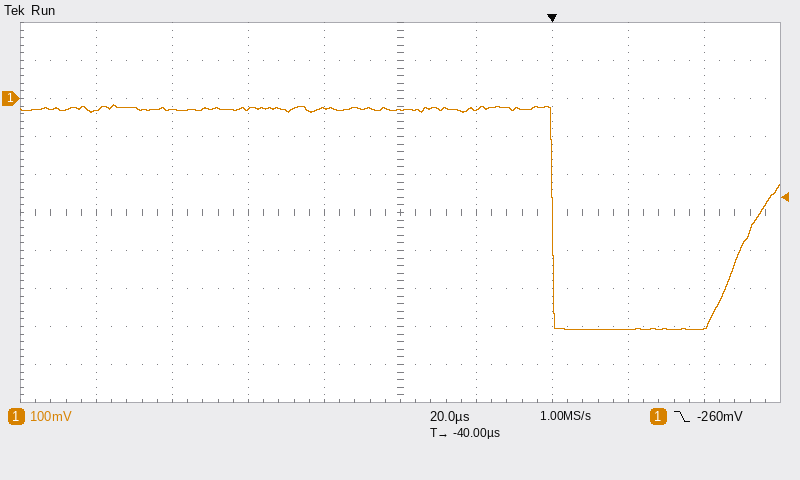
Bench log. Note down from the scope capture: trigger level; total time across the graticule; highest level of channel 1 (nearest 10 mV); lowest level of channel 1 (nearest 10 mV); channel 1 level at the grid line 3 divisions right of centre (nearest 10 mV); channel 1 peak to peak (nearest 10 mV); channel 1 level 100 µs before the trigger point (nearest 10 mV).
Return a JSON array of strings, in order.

["-260 mV", "200 µs", "-20 mV", "-610 mV", "-610 mV", "590 mV", "-30 mV"]
